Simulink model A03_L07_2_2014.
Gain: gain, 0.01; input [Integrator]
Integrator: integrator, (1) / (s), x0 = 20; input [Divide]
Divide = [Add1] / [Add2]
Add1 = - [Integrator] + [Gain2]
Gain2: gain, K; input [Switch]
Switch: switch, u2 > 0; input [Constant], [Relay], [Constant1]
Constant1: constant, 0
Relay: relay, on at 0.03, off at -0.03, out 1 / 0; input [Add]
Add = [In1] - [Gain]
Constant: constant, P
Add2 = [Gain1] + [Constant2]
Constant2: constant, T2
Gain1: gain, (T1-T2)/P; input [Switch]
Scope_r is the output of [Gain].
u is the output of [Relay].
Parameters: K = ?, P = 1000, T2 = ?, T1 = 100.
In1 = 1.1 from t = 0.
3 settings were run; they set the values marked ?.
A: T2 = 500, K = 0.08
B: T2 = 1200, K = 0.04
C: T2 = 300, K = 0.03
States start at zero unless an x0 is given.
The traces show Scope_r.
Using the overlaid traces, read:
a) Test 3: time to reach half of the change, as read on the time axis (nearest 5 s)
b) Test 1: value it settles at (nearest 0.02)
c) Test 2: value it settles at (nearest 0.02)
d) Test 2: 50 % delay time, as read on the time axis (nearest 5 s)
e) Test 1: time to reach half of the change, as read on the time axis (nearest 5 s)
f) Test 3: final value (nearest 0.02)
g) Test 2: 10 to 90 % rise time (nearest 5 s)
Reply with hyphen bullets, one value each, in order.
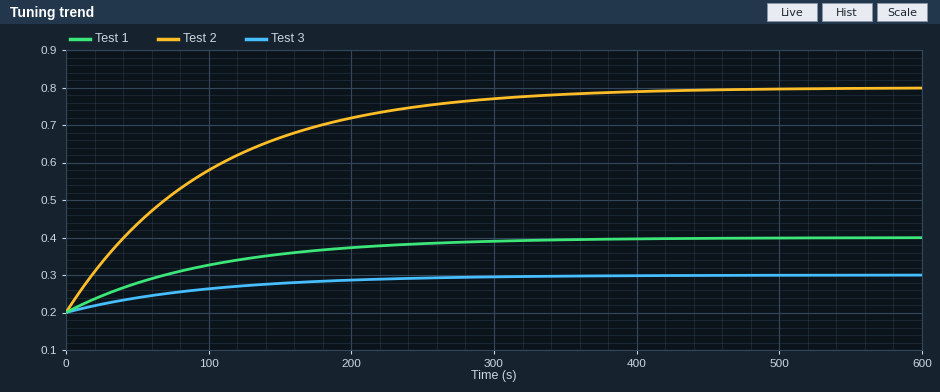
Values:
- 70 s
- 0.40
- 0.80
- 70 s
- 70 s
- 0.30
- 220 s
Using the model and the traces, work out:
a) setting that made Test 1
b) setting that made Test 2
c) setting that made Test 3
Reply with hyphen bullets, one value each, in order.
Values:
- B
- A
- C
